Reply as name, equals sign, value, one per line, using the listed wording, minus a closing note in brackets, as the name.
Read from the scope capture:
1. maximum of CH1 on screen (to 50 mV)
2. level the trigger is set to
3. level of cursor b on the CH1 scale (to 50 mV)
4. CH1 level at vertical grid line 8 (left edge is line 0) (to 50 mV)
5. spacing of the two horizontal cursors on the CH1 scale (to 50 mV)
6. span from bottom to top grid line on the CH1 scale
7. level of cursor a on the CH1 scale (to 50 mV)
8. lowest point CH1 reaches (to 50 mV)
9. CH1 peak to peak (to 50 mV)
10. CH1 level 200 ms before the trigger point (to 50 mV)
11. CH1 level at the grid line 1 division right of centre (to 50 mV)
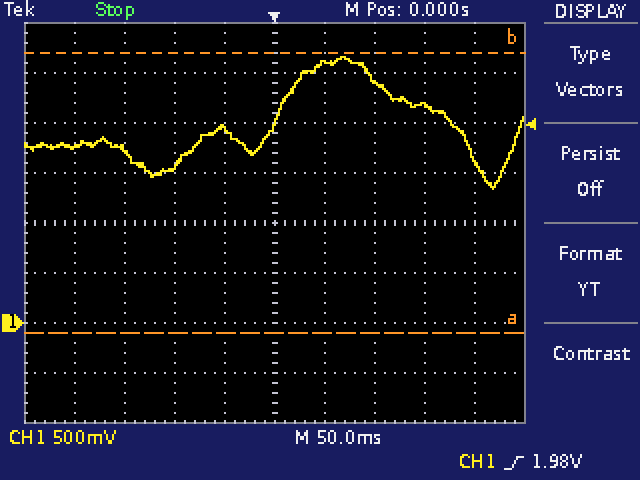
maximum of CH1 on screen = 2.65 V
level the trigger is set to = 1.98 V
level of cursor b on the CH1 scale = 2.70 V
CH1 level at vertical grid line 8 (left edge is line 0) = 2.20 V
spacing of the two horizontal cursors on the CH1 scale = 2.80 V
span from bottom to top grid line on the CH1 scale = 4 V
level of cursor a on the CH1 scale = -100 mV
lowest point CH1 reaches = 1.35 V
CH1 peak to peak = 1.30 V
CH1 level 200 ms before the trigger point = 1.75 V
CH1 level at the grid line 1 division right of centre = 2.60 V
